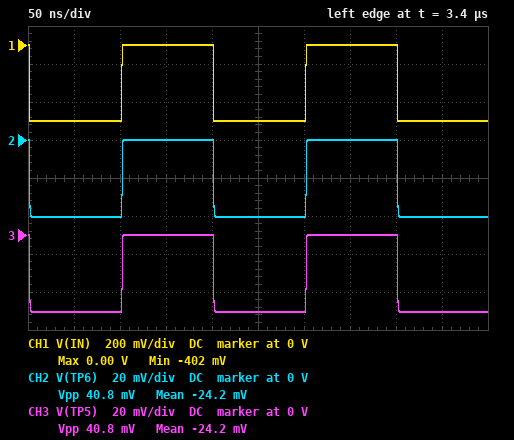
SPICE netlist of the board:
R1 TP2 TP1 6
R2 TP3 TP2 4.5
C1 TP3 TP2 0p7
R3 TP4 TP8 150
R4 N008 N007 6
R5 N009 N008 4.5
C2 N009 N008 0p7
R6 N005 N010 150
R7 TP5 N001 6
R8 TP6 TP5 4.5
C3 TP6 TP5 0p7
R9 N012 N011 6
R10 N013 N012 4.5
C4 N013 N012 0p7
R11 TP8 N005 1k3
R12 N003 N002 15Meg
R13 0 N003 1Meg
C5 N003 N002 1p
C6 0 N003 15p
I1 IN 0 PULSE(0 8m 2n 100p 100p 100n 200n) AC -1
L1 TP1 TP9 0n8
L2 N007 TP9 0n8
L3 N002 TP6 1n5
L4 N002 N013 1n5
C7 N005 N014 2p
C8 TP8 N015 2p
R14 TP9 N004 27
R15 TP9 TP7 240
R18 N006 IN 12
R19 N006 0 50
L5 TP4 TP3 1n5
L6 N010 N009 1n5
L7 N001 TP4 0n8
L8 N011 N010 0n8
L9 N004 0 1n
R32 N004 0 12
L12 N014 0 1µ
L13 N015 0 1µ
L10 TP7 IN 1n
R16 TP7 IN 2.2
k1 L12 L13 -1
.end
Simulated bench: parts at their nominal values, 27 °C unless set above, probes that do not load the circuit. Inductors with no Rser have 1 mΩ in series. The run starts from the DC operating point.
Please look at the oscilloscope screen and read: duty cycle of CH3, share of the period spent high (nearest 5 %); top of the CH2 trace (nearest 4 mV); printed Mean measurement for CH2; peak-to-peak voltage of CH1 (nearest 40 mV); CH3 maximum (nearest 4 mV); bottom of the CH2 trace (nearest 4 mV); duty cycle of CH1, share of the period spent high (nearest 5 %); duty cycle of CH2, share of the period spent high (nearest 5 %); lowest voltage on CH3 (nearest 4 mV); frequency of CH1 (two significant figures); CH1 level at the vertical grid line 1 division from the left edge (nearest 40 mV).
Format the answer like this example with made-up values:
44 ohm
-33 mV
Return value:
50 %
0 V
-24.2 mV
400 mV
0 V
-40 mV
50 %
50 %
-40 mV
5.0 MHz
-400 mV
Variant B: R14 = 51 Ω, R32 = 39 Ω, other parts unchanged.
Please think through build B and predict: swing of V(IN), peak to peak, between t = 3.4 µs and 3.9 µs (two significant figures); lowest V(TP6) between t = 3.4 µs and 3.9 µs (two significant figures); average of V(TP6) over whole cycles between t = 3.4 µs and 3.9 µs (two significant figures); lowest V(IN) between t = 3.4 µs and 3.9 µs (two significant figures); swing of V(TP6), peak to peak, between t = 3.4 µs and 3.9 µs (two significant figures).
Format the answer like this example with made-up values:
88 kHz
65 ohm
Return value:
410 mV
-72 mV
-36 mV
-410 mV
72 mV
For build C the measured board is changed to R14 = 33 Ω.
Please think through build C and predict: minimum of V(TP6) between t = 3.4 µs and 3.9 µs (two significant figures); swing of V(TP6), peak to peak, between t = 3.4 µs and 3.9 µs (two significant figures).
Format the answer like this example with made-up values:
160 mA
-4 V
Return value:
-49 mV
49 mV
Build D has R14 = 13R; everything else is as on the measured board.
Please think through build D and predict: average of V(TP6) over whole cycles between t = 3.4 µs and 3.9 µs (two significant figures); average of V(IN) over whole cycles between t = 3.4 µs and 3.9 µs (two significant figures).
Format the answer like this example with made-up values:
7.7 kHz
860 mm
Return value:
-10 mV
-200 mV
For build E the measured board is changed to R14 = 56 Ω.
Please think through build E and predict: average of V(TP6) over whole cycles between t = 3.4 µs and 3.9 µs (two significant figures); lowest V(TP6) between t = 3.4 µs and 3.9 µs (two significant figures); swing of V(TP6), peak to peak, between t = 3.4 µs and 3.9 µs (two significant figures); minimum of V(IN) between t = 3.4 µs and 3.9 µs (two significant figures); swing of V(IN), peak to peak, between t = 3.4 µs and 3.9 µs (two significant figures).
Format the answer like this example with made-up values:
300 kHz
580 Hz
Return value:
-39 mV
-78 mV
78 mV
-410 mV
410 mV
